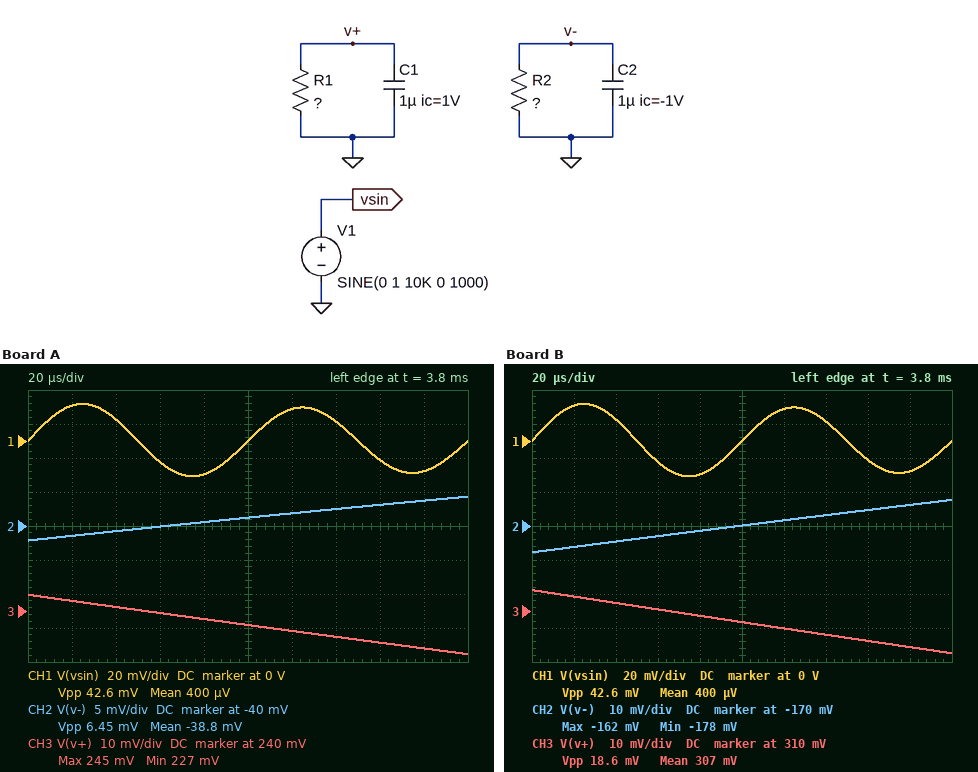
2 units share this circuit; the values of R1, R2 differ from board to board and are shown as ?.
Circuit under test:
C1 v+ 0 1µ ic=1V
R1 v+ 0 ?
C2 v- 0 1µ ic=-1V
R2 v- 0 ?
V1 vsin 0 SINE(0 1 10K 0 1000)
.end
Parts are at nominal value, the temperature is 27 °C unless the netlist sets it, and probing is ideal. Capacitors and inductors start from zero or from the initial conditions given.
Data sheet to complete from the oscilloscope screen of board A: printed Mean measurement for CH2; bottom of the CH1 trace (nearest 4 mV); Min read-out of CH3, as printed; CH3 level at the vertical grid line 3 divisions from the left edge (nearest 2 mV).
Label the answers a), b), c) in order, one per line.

a) -38.8 mV
b) -20 mV
c) 227 mV
d) 240 mV
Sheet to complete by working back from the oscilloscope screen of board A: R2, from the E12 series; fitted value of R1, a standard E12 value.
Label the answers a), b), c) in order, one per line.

a) 1.2 kΩ
b) 2.7 kΩ
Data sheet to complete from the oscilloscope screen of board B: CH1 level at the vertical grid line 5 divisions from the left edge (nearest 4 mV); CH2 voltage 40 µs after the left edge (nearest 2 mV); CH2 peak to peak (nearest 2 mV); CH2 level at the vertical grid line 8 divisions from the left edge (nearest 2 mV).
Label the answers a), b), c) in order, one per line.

a) 0 V
b) -174 mV
c) 16 mV
d) -166 mV
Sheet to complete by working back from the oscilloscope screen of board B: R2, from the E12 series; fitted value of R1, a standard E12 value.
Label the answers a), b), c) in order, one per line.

a) 2.2 kΩ
b) 3.3 kΩ
